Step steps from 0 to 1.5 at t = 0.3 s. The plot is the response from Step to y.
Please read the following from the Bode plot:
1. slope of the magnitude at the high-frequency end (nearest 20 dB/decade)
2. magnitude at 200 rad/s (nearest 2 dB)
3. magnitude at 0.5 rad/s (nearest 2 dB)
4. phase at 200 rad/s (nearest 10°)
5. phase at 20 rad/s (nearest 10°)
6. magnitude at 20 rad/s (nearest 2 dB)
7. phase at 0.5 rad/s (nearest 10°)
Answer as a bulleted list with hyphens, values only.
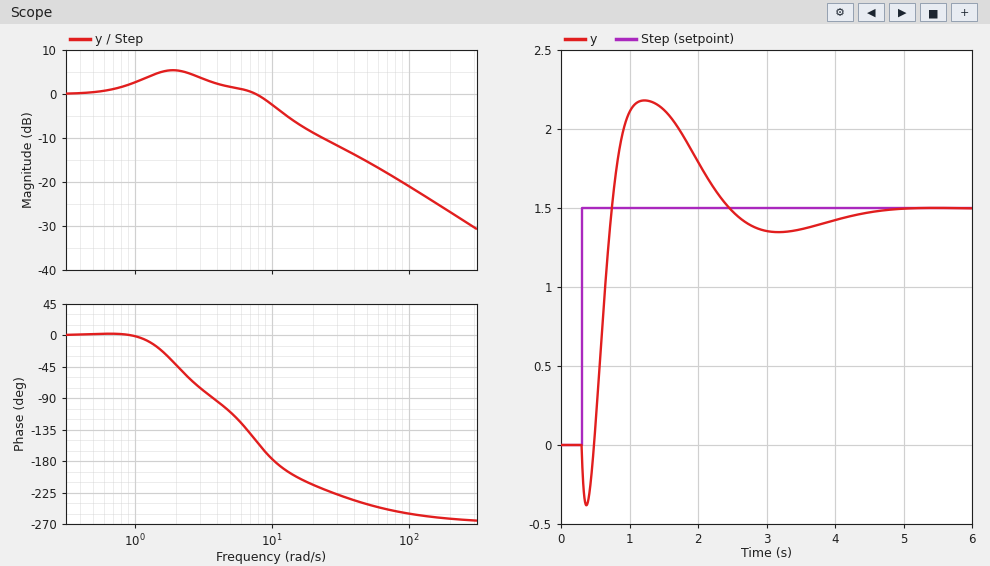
- -20 dB/decade
- -26 dB
- 0 dB
- -260°
- -210°
- -8 dB
- 0°
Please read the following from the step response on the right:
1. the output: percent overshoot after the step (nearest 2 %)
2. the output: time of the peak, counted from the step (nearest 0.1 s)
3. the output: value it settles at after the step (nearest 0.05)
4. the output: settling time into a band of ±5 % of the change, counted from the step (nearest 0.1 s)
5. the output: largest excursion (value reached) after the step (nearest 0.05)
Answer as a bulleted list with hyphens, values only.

- 46 %
- 0.9 s
- 1.50
- 3.7 s
- 2.20
